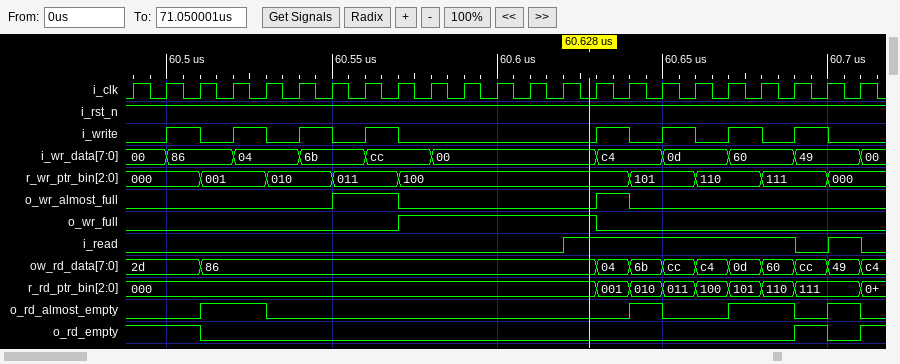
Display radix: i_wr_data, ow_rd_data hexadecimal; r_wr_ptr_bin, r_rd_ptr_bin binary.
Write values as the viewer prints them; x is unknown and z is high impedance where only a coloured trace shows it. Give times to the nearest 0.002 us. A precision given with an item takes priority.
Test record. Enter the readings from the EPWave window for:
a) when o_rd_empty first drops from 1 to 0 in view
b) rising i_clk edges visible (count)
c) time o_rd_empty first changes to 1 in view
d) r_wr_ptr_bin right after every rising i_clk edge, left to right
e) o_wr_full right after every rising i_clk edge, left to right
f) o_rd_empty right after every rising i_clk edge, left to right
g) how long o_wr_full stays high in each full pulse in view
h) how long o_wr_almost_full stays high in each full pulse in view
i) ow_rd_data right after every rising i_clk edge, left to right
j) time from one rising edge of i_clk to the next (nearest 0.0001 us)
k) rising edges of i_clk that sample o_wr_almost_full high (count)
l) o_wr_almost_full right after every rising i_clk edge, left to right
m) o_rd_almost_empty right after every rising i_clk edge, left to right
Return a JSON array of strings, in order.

["60.51 us", "23", "60.69 us", "000, 000, 001, 001, 010, 010, 011, 011, 100, 100, 100, 100, 100, 100, 100, 101, 101, 110, 110, 111, 111, 000, 000", "0 0 0 0 0 0 0 0 1 1 1 1 1 1 0 0 0 0 0 0 0 0 0", "1 1 0 0 0 0 0 0 0 0 0 0 0 0 0 0 0 0 0 0 1 0 1", "0.06 us", "0.02 us, 0.01 us", "2d, 2d, 86, 86, 86, 86, 86, 86, 86, 86, 86, 86, 86, 86, 04, 6b, cc, c4, 0d, 60, cc, 49, c4", "0.01 us", "3", "0 0 0 0 0 0 1 1 0 0 0 0 0 0 1 0 0 0 0 0 0 0 0", "0 0 1 1 0 0 0 0 0 0 0 0 0 0 0 1 0 0 1 1 0 1 0"]
